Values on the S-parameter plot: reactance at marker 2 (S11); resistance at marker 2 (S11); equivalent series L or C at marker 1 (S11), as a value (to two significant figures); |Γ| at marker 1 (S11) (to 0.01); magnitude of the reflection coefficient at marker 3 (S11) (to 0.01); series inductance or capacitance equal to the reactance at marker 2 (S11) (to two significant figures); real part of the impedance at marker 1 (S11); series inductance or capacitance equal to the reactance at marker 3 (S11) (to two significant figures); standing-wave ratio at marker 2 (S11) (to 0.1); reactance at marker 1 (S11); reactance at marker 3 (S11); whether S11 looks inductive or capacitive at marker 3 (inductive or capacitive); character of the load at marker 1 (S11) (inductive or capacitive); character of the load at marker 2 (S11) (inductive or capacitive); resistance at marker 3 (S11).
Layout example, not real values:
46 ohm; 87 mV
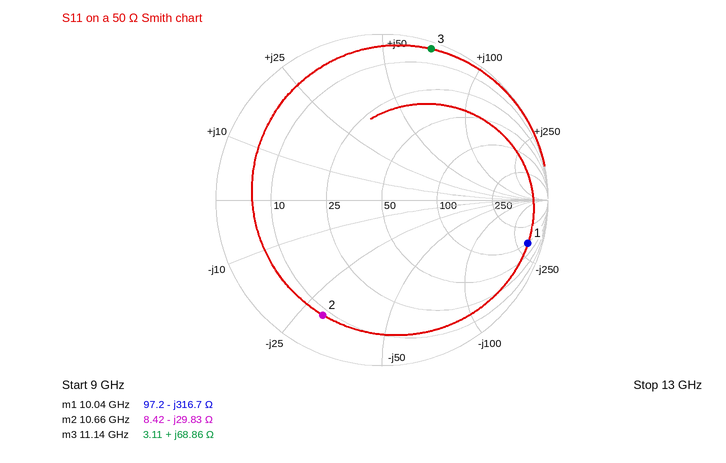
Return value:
-29.83 Ω; 8.42 Ω; 50 fF; 0.92; 0.96; 500 fF; 97.2 Ω; 980 pH; 8.1; -316.7 Ω; +68.86 Ω; inductive; capacitive; capacitive; 3.11 Ω
